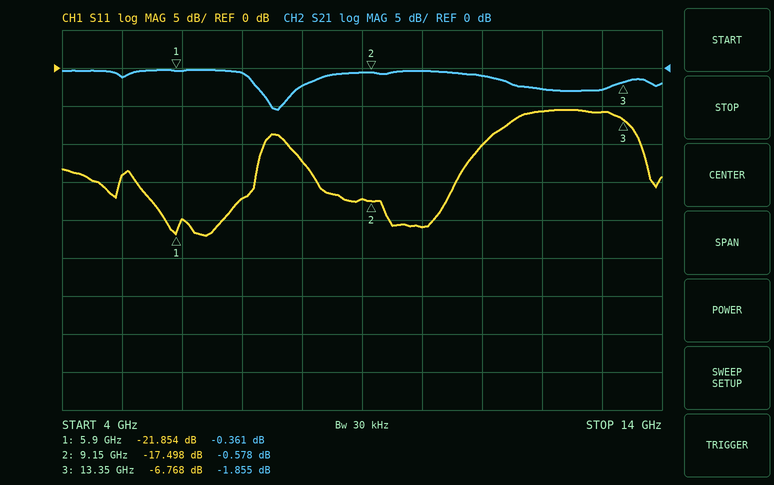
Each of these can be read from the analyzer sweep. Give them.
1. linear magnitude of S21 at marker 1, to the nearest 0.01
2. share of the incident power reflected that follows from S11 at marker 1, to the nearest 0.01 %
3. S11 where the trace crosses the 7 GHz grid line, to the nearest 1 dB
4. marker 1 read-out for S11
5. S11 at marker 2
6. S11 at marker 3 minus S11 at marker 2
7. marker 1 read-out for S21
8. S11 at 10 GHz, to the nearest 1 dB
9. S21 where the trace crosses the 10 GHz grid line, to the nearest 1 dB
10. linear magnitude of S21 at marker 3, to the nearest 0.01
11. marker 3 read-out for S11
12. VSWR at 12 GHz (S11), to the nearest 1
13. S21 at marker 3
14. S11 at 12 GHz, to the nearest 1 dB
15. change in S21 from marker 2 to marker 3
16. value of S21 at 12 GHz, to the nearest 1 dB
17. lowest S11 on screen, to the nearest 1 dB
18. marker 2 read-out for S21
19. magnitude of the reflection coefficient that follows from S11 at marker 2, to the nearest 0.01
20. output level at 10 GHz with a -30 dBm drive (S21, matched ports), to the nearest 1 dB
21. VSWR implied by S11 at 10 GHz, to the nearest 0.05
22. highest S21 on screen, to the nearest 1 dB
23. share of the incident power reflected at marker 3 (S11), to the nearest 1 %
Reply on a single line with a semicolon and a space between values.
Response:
0.96; 0.65 %; -17 dB; -21.854 dB; -17.498 dB; 10.730 dB; -0.361 dB; -21 dB; 0 dB; 0.81; -6.768 dB; 3; -1.855 dB; -6 dB; -1.277 dB; -3 dB; -22 dB; -0.578 dB; 0.13; -30 dBm; 1.20; 0 dB; 21 %
